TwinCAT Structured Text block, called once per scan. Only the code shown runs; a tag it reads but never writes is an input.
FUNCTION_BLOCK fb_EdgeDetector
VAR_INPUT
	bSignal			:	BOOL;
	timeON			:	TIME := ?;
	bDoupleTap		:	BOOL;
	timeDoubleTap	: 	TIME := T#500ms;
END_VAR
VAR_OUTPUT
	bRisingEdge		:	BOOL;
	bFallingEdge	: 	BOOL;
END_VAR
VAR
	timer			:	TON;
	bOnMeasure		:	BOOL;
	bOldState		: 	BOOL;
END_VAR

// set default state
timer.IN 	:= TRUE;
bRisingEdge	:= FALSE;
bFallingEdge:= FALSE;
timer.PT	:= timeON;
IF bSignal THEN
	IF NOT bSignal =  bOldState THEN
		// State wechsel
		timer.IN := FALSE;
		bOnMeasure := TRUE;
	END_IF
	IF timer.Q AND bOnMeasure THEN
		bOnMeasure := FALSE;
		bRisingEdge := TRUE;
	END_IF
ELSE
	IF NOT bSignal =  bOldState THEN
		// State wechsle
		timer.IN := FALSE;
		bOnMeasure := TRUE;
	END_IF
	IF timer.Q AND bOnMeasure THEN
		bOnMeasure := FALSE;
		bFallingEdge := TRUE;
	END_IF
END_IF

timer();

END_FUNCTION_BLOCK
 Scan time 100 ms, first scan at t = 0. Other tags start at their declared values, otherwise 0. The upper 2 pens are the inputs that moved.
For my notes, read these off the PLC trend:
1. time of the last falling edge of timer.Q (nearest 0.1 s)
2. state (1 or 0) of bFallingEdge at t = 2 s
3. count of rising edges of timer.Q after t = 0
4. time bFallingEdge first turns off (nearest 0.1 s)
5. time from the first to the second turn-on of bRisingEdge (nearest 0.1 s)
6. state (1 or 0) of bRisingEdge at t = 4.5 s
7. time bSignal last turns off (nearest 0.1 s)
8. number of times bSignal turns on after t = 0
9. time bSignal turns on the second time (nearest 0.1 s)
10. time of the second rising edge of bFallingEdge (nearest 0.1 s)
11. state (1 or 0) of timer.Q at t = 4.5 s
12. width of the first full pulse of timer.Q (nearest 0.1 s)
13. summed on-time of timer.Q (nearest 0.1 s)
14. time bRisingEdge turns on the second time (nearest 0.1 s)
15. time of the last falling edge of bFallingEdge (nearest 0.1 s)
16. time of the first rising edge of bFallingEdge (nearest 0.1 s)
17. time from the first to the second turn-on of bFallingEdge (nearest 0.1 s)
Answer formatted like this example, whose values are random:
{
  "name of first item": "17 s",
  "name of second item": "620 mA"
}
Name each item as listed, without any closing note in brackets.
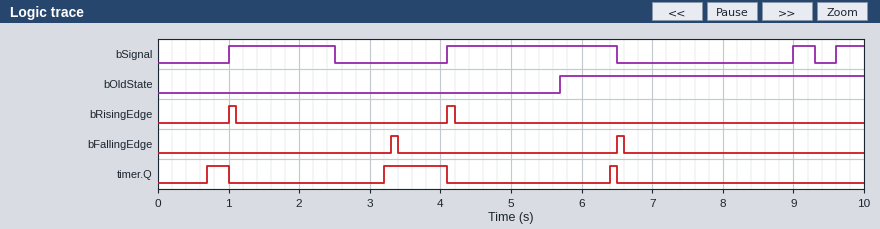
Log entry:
{
  "time of the last falling edge of timer.Q": "6.5 s",
  "state (1 or 0) of bFallingEdge at t = 2 s": "0",
  "count of rising edges of timer.Q after t = 0": "3",
  "time bFallingEdge first turns off": "3.4 s",
  "time from the first to the second turn-on of bRisingEdge": "3.1 s",
  "state (1 or 0) of bRisingEdge at t = 4.5 s": "0",
  "time bSignal last turns off": "9.3 s",
  "number of times bSignal turns on after t = 0": "4",
  "time bSignal turns on the second time": "4.1 s",
  "time of the second rising edge of bFallingEdge": "6.5 s",
  "state (1 or 0) of timer.Q at t = 4.5 s": "0",
  "width of the first full pulse of timer.Q": "0.3 s",
  "summed on-time of timer.Q": "1.3 s",
  "time bRisingEdge turns on the second time": "4.1 s",
  "time of the last falling edge of bFallingEdge": "6.6 s",
  "time of the first rising edge of bFallingEdge": "3.3 s",
  "time from the first to the second turn-on of bFallingEdge": "3.2 s"
}
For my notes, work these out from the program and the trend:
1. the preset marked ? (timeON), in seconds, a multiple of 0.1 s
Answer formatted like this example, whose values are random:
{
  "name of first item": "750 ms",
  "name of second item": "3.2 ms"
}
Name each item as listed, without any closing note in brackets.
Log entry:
{
  "the preset marked ? (timeON), in seconds, a multiple of 0.1 s": "0.7 s"
}
